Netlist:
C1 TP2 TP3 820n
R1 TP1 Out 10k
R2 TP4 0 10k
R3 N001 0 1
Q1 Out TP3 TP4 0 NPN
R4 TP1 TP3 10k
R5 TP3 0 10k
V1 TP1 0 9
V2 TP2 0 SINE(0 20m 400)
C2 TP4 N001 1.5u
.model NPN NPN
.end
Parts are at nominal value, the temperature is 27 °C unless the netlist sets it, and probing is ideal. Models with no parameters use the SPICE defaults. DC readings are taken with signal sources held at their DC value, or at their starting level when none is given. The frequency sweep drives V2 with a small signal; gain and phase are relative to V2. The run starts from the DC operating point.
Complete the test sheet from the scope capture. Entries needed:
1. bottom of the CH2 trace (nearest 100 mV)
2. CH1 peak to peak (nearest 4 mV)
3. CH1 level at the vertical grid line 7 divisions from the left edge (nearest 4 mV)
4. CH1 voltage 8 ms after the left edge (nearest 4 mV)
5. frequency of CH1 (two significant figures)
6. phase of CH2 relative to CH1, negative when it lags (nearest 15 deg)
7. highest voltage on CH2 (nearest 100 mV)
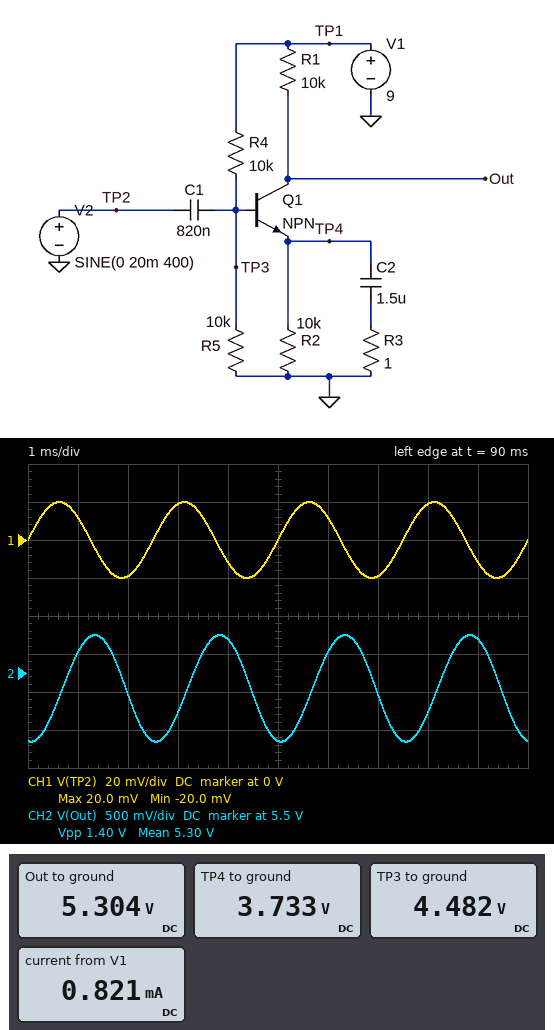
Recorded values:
4.6 V
40 mV
-20 mV
20 mV
400 Hz
-105 deg
6.0 V
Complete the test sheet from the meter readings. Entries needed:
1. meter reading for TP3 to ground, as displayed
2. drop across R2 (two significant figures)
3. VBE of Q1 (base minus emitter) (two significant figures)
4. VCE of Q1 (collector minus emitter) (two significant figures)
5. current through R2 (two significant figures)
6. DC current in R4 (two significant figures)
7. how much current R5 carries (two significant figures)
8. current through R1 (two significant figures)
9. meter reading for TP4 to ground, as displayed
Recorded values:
4.482 V
3.7 V
750 mV
1.6 V
370 µA
450 µA
450 µA
370 µA
3.733 V
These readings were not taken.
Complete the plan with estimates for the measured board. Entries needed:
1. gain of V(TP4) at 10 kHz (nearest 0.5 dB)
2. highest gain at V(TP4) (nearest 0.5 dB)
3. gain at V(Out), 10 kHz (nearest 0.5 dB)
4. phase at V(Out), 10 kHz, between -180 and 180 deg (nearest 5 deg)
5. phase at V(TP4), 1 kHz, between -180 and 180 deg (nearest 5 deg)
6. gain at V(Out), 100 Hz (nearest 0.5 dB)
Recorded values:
-16.5 dB
-0.5 dB
43.0 dB
-170 deg
-30 deg
18.5 dB
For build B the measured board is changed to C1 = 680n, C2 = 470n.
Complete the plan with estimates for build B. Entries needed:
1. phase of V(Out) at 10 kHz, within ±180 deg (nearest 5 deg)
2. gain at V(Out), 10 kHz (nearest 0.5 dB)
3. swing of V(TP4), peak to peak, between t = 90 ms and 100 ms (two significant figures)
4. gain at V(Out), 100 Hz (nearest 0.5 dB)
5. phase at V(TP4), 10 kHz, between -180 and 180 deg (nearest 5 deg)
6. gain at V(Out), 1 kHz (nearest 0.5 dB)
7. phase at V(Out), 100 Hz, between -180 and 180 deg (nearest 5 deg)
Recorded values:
-155 deg
42.0 dB
39 mV
9.0 dB
-60 deg
29.0 dB
-85 deg
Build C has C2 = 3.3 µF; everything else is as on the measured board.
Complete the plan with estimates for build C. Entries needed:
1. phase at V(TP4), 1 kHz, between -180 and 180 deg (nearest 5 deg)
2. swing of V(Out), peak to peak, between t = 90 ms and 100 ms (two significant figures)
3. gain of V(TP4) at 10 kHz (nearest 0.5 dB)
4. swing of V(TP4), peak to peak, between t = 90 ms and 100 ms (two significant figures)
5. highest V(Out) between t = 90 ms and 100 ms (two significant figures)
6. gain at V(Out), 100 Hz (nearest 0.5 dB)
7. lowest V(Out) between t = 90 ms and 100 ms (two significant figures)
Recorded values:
-50 deg
2.7 V
-23.0 dB
33 mV
6.6 V
25.0 dB
3.9 V
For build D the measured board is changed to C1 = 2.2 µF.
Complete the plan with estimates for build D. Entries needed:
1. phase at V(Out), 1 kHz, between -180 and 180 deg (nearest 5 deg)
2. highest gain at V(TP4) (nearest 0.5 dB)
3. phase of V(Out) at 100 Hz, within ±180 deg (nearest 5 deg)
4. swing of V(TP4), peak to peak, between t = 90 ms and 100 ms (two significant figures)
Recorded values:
-125 deg
0 dB
-90 deg
38 mV
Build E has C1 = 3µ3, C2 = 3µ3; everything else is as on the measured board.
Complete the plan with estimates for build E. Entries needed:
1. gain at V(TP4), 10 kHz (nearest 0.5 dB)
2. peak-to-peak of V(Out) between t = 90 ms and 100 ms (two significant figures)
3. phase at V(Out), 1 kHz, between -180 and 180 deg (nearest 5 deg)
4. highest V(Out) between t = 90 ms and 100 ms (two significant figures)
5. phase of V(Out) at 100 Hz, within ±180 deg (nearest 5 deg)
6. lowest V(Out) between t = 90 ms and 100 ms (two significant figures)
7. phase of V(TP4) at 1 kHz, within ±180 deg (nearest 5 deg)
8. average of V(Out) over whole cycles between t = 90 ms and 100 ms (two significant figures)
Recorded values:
-23.0 dB
2.7 V
-145 deg
6.6 V
-95 deg
3.9 V
-55 deg
5.3 V
